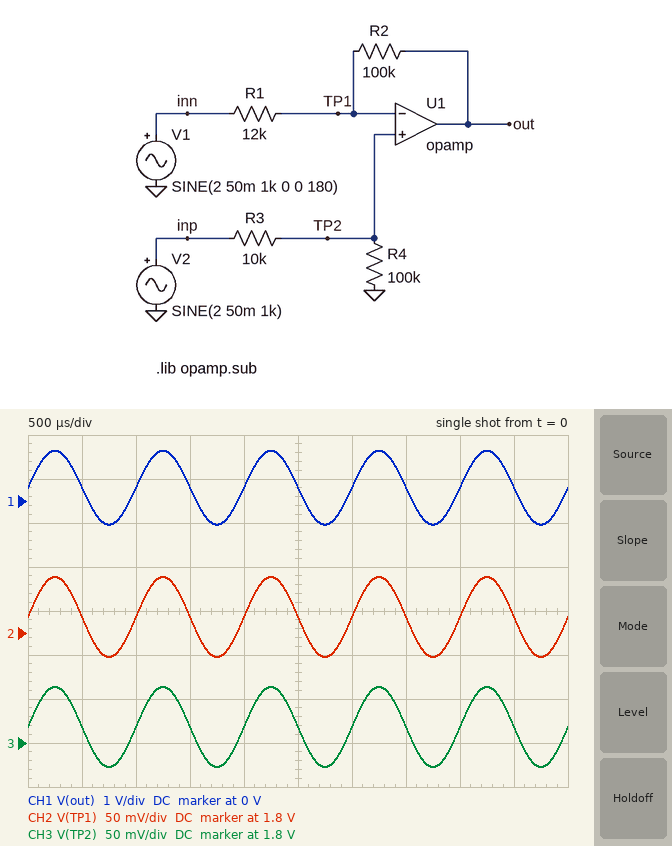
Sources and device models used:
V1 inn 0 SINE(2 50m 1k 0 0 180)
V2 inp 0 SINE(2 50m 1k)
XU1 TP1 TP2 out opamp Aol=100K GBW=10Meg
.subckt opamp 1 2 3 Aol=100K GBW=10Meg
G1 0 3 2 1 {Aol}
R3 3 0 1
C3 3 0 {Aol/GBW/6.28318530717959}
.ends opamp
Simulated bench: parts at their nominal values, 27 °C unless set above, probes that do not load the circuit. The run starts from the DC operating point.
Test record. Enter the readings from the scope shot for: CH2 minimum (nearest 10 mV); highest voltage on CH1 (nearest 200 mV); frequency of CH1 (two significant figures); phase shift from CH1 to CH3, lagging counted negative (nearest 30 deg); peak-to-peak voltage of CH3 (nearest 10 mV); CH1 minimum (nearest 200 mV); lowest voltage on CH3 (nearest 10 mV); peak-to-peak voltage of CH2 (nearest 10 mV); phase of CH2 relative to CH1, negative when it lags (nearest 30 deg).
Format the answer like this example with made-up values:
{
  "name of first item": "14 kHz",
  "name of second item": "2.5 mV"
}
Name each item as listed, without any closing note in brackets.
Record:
{
  "CH2 minimum": "1.77 V",
  "highest voltage on CH1": "1.2 V",
  "frequency of CH1": "1.0 kHz",
  "phase shift from CH1 to CH3, lagging counted negative": "0 deg",
  "peak-to-peak voltage of CH3": "90 mV",
  "CH1 minimum": "-600 mV",
  "lowest voltage on CH3": "1.77 V",
  "peak-to-peak voltage of CH2": "90 mV",
  "phase of CH2 relative to CH1, negative when it lags": "0 deg"
}
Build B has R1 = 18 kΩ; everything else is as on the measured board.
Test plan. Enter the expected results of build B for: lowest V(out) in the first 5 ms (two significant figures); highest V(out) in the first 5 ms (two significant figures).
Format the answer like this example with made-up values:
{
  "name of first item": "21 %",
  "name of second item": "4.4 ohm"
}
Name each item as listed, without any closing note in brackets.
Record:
{
  "lowest V(out) in the first 5 ms": "230 mV",
  "highest V(out) in the first 5 ms": "1.4 V"
}
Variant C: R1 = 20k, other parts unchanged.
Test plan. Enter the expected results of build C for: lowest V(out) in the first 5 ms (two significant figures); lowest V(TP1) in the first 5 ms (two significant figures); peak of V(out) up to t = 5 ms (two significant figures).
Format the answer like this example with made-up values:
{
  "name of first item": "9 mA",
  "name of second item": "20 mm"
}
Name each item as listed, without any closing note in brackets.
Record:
{
  "lowest V(out) in the first 5 ms": "390 mV",
  "lowest V(TP1) in the first 5 ms": "1.8 V",
  "peak of V(out) up to t = 5 ms": "1.4 V"
}
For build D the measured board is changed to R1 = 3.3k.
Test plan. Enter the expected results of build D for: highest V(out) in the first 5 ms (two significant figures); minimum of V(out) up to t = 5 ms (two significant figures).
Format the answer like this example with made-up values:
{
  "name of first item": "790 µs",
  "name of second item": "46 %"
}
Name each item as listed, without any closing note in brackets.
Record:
{
  "highest V(out) in the first 5 ms": "-750 mV",
  "minimum of V(out) up to t = 5 ms": "-6.6 V"
}
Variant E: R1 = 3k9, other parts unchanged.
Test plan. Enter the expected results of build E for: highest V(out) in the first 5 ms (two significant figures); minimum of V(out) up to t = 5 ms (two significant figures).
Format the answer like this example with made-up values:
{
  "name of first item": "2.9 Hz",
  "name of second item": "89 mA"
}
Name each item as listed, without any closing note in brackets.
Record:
{
  "highest V(out) in the first 5 ms": "-350 mV",
  "minimum of V(out) up to t = 5 ms": "-5.3 V"
}
